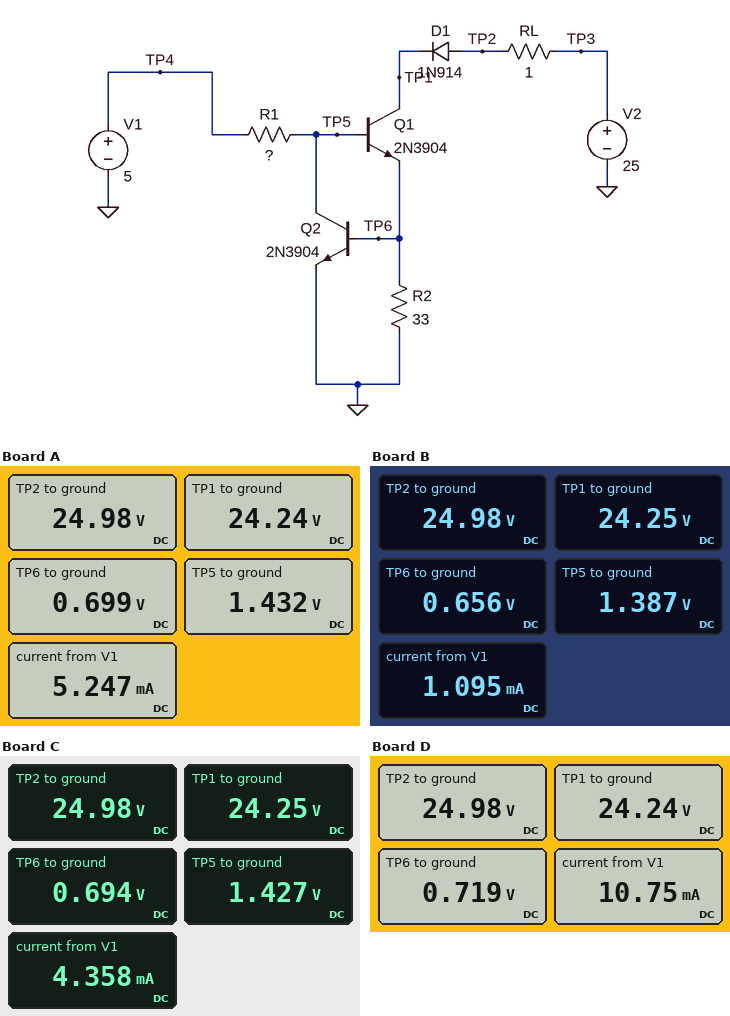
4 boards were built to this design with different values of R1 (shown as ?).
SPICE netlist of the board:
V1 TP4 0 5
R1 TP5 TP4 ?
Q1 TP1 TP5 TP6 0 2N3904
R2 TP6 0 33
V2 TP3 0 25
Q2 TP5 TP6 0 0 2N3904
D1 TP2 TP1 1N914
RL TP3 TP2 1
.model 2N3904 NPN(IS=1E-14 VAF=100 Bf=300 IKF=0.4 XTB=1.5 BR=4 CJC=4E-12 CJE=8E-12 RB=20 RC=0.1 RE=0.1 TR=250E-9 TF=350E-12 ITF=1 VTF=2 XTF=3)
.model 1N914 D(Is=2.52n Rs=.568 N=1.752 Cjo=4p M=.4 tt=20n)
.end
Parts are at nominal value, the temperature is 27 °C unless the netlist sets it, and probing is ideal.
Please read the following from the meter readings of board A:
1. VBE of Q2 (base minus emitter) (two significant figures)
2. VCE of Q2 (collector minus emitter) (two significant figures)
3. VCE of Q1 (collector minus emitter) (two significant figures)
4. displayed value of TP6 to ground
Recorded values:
700 mV
1.4 V
24 V
0.699 V
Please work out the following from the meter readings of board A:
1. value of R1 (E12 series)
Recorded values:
680 Ω
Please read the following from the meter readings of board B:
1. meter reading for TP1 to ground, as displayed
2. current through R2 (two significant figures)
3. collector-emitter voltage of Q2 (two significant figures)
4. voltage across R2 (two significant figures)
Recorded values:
24.25 V
20 mA
1.4 V
660 mV
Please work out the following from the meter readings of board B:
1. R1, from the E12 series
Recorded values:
3.3 kΩ
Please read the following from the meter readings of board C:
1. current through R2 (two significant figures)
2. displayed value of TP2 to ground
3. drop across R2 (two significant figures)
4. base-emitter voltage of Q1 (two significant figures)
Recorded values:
21 mA
24.98 V
690 mV
730 mV
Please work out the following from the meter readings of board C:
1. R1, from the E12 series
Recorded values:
820 Ω
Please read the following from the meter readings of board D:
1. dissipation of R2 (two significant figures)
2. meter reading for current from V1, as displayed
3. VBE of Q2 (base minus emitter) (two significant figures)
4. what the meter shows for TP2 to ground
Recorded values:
16 mW
10.75 mA
720 mV
24.98 V
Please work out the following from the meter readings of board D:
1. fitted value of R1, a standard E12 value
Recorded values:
330 Ω
